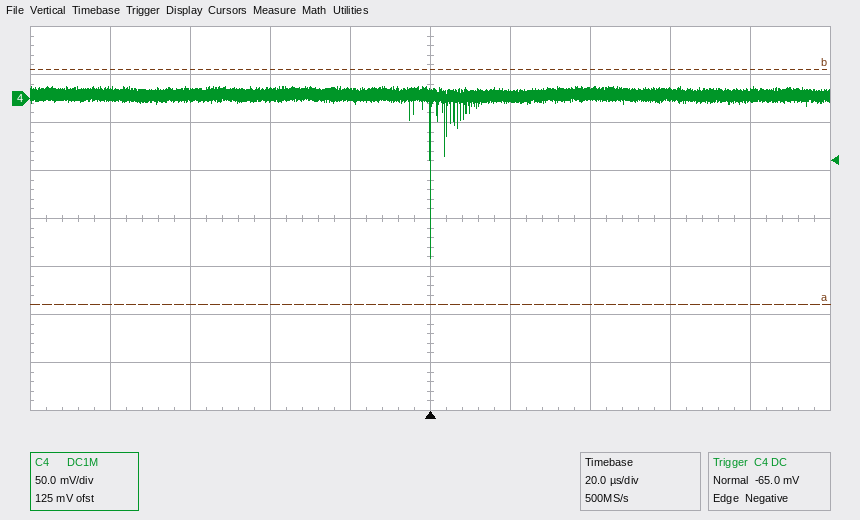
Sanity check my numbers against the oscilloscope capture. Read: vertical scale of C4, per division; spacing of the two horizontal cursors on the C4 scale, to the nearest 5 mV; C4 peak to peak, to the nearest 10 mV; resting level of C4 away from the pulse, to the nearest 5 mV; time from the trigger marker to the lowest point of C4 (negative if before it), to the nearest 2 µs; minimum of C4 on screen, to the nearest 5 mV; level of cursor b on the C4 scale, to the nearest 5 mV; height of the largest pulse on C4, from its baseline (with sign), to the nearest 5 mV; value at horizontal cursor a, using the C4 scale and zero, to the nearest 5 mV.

50 mV
245 mV
180 mV
5 mV
0 µs
-165 mV
30 mV
-170 mV
-215 mV
